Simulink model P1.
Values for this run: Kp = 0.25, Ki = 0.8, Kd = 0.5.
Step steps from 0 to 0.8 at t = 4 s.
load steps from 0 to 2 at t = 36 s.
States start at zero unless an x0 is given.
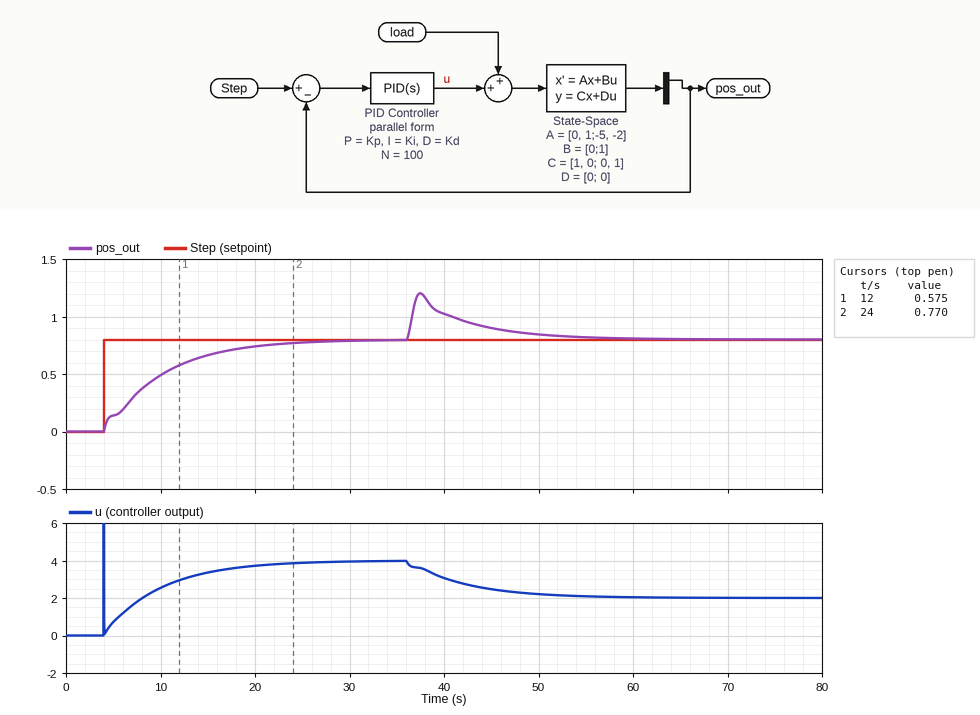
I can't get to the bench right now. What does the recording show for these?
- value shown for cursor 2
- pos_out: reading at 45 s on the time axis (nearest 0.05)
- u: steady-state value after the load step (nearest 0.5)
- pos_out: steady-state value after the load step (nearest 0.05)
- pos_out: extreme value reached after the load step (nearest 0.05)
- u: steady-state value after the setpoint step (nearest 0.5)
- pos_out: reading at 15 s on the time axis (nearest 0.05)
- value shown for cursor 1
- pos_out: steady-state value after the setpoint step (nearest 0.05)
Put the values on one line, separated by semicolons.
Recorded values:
0.770; 0.90; 2.0; 0.80; 1.20; 4.0; 0.65; 0.575; 0.80
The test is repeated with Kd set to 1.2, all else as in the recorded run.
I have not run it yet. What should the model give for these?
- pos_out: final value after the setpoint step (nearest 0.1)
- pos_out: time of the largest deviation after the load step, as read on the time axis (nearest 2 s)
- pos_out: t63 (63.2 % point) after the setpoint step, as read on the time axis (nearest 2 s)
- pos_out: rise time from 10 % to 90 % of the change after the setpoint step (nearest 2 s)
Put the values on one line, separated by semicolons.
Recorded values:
0.8; 38 s; 10 s; 14 s
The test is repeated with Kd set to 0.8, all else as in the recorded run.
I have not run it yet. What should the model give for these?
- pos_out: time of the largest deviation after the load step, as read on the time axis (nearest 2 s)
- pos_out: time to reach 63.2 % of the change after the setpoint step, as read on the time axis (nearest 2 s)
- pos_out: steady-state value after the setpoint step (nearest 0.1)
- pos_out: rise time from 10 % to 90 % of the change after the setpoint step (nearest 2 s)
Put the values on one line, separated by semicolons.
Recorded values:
38 s; 10 s; 0.8; 14 s
